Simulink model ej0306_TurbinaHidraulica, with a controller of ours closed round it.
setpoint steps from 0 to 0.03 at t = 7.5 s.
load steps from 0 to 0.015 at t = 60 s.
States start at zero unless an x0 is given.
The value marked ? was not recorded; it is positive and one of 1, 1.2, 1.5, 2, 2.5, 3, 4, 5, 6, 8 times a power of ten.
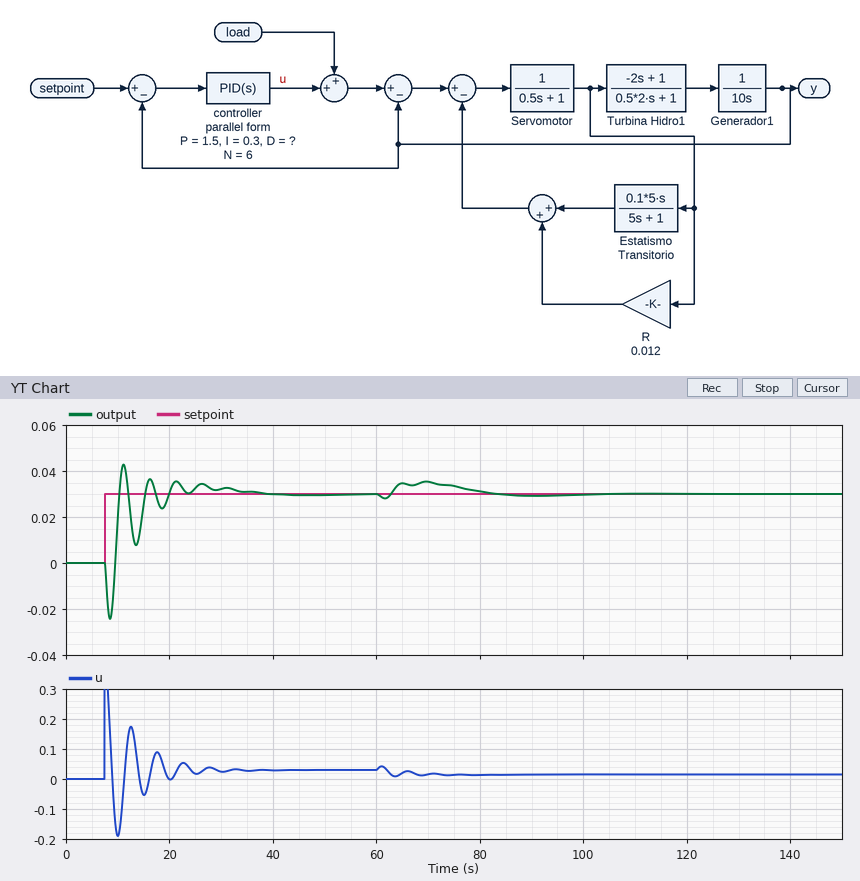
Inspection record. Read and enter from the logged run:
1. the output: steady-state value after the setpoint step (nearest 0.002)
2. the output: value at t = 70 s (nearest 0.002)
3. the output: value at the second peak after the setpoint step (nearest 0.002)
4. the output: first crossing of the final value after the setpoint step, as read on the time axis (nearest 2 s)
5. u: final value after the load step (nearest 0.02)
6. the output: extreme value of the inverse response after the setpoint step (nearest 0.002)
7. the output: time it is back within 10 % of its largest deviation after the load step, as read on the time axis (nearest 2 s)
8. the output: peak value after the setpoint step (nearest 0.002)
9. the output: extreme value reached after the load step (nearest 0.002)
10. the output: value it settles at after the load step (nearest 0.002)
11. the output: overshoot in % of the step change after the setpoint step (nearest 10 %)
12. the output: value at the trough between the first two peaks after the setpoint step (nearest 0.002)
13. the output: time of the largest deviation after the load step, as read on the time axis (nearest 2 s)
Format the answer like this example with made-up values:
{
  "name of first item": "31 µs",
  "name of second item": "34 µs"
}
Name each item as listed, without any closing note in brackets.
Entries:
{
  "the output: steady-state value after the setpoint step": "0.030",
  "the output: value at t = 70 s": "0.036",
  "the output: value at the second peak after the setpoint step": "0.036",
  "the output: first crossing of the final value after the setpoint step, as read on the time axis": "10 s",
  "u: final value after the load step": "0.02",
  "the output: extreme value of the inverse response after the setpoint step": "-0.024",
  "the output: time it is back within 10 % of its largest deviation after the load step, as read on the time axis": "96 s",
  "the output: peak value after the setpoint step": "0.042",
  "the output: extreme value reached after the load step": "0.036",
  "the output: value it settles at after the load step": "0.030",
  "the output: overshoot in % of the step change after the setpoint step": "40 %",
  "the output: value at the trough between the first two peaks after the setpoint step": "0.008",
  "the output: time of the largest deviation after the load step, as read on the time axis": "70 s"
}
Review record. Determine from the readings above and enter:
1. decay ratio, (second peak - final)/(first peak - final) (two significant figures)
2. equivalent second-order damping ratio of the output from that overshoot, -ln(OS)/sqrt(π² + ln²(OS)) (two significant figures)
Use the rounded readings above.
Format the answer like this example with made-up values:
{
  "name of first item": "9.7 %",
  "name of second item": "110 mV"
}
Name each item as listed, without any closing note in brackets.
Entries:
{
  "decay ratio, (second peak - final)/(first peak - final)": "0.50",
  "equivalent second-order damping ratio of the output from that overshoot, -ln(OS)/sqrt(π² + ln²(OS))": "0.28"
}
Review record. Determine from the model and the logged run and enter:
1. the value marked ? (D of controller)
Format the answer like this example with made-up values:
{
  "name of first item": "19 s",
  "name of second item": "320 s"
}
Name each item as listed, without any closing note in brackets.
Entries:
{
  "the value marked ?": "6"
}
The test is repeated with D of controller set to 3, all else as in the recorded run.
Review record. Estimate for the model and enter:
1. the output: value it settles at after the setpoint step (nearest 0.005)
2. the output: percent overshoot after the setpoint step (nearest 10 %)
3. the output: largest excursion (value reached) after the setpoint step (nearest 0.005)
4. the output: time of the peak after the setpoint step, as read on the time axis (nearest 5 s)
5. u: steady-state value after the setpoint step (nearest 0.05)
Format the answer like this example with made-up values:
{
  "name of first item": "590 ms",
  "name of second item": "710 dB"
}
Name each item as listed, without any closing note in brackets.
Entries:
{
  "the output: value it settles at after the setpoint step": "0.030",
  "the output: percent overshoot after the setpoint step": "20 %",
  "the output: largest excursion (value reached) after the setpoint step": "0.035",
  "the output: time of the peak after the setpoint step, as read on the time axis": "20 s",
  "u: steady-state value after the setpoint step": "0.05"
}
